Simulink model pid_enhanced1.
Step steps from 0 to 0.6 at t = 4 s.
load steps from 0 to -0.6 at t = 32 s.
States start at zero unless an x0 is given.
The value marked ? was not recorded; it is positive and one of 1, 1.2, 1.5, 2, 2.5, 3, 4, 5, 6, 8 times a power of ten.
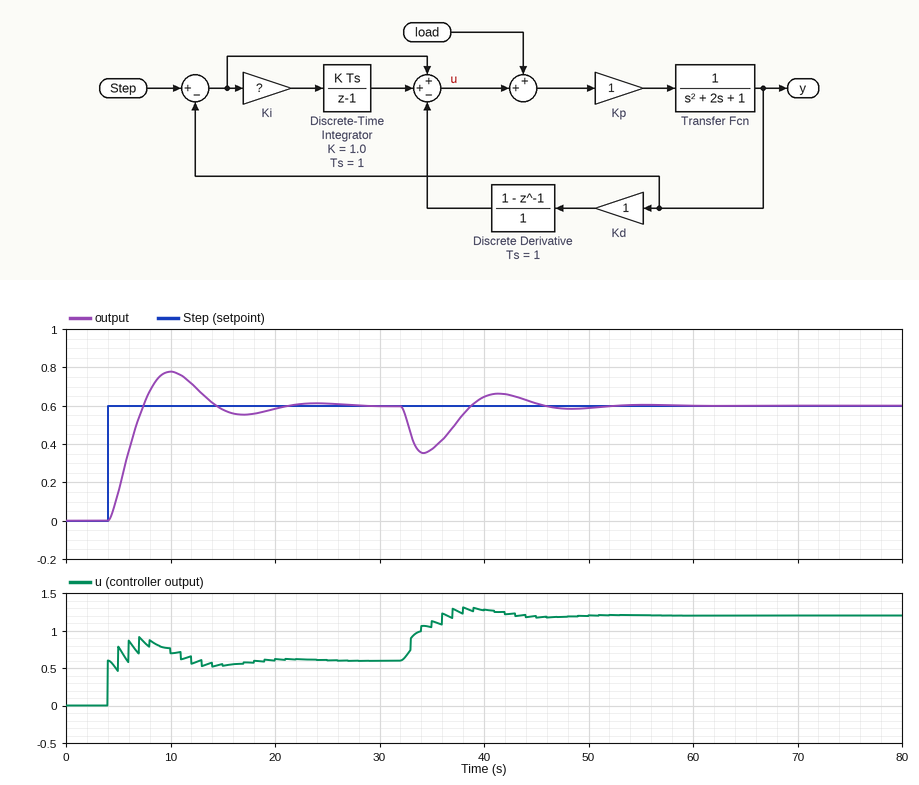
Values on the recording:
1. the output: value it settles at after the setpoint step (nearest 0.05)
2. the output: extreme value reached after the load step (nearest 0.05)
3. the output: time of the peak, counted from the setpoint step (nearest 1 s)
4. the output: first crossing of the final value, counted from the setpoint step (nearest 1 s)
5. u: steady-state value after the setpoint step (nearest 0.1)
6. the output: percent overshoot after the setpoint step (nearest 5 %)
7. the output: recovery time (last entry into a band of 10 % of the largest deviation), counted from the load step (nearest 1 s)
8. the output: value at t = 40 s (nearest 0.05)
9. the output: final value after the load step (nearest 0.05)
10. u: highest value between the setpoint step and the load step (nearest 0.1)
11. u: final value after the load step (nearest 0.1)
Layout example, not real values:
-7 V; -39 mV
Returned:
0.60; 0.35; 6 s; 3 s; 0.6; 30 %; 12 s; 0.65; 0.60; 0.9; 1.2
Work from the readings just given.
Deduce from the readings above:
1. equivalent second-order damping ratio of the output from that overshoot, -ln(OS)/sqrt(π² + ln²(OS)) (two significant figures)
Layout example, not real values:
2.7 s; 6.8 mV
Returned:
0.36
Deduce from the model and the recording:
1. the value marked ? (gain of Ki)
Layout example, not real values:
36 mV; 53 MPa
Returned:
0.8
